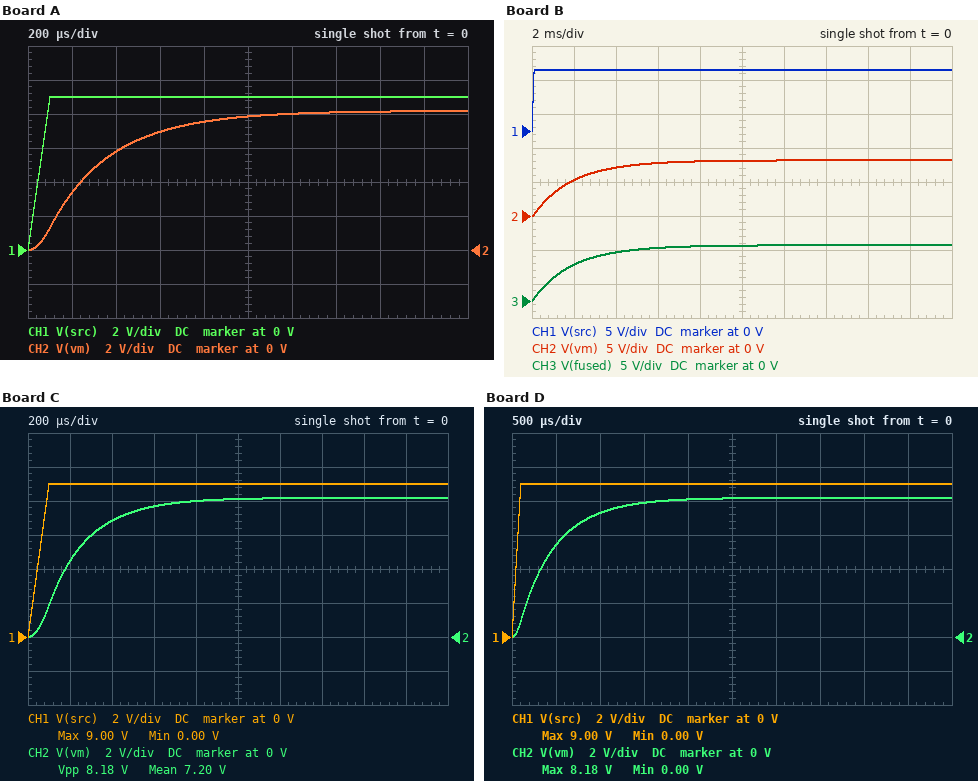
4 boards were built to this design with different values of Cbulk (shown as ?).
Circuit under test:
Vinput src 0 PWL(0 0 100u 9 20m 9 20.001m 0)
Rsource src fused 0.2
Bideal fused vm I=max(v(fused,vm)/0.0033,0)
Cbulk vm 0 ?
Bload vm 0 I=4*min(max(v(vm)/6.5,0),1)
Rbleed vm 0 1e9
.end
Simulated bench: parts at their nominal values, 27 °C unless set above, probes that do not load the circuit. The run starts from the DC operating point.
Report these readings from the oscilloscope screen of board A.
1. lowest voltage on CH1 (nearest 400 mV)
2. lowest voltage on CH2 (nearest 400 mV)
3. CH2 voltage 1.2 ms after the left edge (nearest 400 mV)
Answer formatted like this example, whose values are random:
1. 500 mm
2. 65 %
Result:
1. 0 V
2. 0 V
3. 8.0 V
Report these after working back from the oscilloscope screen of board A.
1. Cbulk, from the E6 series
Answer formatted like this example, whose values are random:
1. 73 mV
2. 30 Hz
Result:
1. 1.5 mF
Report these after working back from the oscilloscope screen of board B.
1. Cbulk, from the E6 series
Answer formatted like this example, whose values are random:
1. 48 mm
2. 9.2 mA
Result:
1. 10 mF
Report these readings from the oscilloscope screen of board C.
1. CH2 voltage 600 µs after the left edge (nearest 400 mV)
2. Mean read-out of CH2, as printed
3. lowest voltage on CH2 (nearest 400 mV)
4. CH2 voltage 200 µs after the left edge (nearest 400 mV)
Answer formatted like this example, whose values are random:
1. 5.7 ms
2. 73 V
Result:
1. 7.6 V
2. 7.20 V
3. 0 V
4. 4.4 V
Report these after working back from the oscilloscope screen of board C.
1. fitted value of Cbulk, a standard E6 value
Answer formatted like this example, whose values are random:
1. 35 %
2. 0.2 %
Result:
1. 1 mF
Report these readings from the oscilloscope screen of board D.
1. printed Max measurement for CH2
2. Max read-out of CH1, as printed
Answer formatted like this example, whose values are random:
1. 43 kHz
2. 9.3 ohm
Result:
1. 8.18 V
2. 9.00 V
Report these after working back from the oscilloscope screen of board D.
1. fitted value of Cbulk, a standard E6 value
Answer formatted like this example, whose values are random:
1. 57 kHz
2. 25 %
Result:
1. 2.2 mF
